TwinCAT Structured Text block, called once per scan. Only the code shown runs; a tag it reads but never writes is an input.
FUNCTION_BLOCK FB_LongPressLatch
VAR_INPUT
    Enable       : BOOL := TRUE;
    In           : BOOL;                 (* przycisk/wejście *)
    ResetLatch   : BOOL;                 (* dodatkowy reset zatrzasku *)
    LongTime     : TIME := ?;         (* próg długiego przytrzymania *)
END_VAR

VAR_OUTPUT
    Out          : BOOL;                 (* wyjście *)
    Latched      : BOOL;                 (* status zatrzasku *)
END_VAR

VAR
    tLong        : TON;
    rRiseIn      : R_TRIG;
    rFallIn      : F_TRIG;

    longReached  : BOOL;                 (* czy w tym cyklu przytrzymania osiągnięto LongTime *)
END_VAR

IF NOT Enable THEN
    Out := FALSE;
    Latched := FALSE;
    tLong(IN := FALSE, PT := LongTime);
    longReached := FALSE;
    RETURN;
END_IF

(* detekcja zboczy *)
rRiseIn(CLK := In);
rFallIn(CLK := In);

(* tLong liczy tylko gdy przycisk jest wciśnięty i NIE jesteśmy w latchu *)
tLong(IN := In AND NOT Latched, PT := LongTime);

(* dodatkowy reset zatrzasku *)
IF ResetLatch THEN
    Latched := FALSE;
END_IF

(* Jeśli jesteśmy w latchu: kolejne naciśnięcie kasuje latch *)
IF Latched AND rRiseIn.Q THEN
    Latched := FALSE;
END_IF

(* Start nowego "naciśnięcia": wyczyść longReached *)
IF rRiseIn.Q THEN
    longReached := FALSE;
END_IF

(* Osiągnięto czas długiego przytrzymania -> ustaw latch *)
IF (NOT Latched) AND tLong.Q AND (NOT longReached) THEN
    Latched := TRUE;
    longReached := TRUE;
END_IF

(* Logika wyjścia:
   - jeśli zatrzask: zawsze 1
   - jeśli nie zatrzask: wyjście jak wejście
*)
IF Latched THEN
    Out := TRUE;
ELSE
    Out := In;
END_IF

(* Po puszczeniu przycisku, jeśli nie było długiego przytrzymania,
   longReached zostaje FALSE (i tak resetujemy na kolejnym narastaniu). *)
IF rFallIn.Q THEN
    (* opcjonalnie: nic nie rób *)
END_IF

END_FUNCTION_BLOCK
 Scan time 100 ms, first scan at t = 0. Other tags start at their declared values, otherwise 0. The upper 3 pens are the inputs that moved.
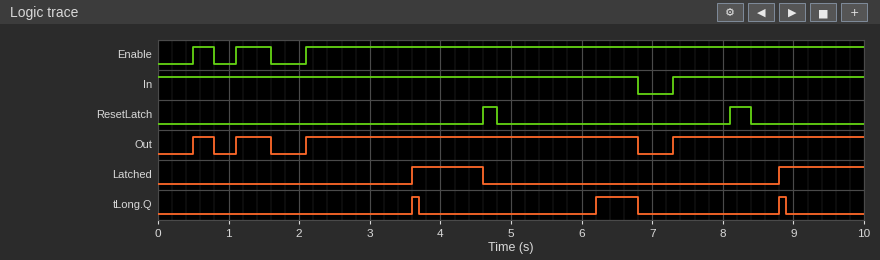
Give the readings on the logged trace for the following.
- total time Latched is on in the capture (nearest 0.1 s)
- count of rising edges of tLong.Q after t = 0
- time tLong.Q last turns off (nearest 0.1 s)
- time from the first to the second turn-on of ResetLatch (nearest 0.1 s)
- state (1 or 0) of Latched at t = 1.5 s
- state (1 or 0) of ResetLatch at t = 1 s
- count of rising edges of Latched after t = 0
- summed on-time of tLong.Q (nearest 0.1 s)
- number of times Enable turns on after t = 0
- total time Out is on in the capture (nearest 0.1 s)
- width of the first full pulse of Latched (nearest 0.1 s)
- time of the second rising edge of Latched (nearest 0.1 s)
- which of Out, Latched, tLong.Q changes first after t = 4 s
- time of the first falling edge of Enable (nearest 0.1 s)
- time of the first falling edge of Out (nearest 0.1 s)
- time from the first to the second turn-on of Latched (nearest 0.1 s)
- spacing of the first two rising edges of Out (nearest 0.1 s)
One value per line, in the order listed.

2.2 s
3
8.9 s
3.5 s
0
0
2
0.8 s
3
8.2 s
1.0 s
8.8 s
Latched
0.8 s
0.8 s
5.2 s
0.6 s
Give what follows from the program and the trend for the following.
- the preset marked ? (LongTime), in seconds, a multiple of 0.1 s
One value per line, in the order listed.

1.5 s
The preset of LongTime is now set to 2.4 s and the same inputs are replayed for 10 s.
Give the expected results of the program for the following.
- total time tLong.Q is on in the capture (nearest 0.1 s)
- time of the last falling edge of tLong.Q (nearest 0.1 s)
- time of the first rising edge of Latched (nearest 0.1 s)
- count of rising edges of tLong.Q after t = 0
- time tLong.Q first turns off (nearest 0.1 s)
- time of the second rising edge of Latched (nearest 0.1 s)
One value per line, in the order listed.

0.2 s
9.8 s
4.5 s
2
4.6 s
9.7 s
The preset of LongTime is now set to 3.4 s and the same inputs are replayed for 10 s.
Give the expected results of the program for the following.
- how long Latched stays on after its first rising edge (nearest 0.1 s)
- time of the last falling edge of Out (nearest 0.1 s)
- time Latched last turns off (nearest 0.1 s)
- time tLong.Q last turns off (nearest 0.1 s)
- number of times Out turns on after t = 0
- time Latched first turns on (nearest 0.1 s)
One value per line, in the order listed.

1.8 s
1.6 s
7.3 s
5.6 s
3
5.5 s
